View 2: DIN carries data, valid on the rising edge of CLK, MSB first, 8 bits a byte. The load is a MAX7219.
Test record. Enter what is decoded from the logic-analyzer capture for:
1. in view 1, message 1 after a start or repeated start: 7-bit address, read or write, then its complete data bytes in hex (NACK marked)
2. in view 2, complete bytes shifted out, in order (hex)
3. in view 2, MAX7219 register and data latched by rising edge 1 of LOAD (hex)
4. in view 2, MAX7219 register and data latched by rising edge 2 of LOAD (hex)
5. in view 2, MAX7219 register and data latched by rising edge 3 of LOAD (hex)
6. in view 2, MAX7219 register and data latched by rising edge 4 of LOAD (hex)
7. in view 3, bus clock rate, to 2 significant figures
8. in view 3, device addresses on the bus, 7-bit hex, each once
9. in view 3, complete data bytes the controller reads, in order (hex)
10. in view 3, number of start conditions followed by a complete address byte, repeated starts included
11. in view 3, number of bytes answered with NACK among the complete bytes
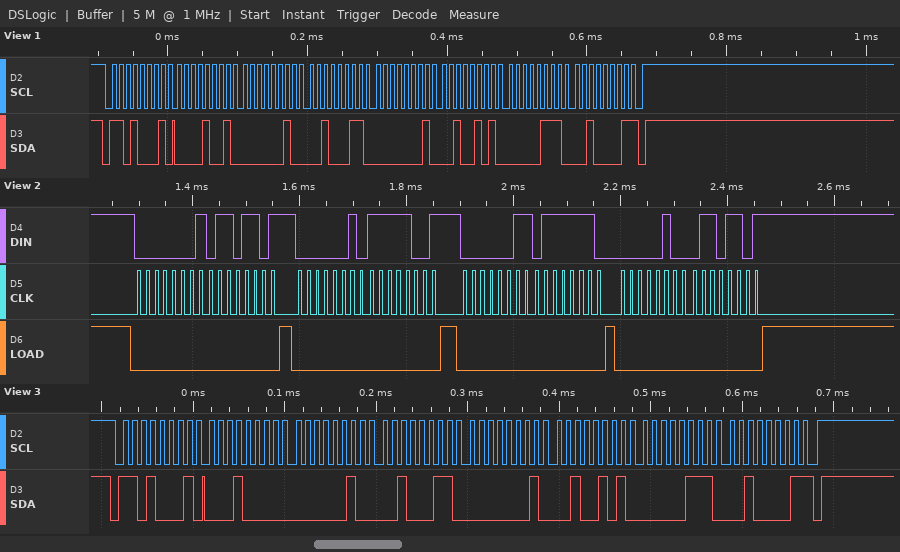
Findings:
0x68 read: 09 02 23 01 25 07 21 NACK
01 6D 02 F9 03 7E 04 6D
register 0x1, data 0x6D
register 0x2, data 0xF9
register 0x3, data 0x7E
register 0x4, data 0x6D
100 kHz
0x68
10 02 23 01 25 07 21
1
1
